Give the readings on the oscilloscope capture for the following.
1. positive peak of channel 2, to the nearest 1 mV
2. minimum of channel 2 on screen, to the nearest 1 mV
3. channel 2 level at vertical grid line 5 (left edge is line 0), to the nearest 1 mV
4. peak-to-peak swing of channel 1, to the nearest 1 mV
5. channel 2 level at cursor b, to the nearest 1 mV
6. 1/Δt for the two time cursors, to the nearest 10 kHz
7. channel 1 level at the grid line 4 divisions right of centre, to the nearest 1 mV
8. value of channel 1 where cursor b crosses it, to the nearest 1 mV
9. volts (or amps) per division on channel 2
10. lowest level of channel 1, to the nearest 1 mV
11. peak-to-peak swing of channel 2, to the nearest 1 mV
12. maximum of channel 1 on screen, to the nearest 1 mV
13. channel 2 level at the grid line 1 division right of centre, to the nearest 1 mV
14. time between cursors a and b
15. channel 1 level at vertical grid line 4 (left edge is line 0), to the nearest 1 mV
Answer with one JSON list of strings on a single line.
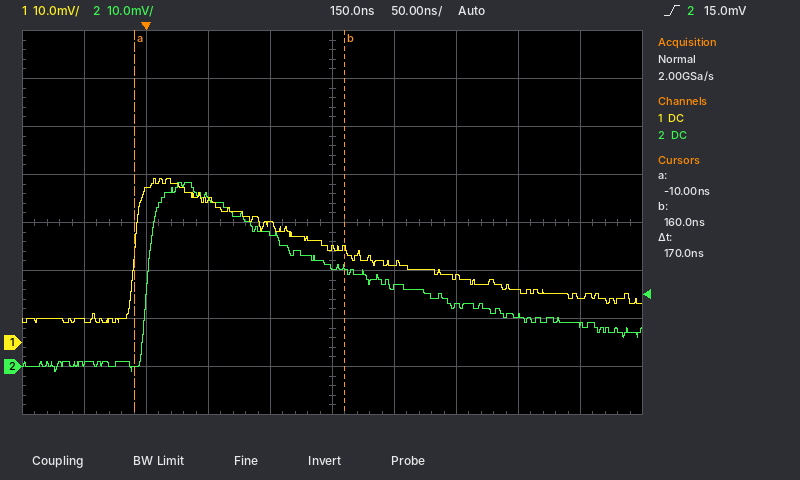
["38 mV", "-1 mV", "21 mV", "30 mV", "20 mV", "5.88 MHz", "9 mV", "19 mV", "10 mV", "4 mV", "39 mV", "34 mV", "17 mV", "170 ns", "25 mV"]
